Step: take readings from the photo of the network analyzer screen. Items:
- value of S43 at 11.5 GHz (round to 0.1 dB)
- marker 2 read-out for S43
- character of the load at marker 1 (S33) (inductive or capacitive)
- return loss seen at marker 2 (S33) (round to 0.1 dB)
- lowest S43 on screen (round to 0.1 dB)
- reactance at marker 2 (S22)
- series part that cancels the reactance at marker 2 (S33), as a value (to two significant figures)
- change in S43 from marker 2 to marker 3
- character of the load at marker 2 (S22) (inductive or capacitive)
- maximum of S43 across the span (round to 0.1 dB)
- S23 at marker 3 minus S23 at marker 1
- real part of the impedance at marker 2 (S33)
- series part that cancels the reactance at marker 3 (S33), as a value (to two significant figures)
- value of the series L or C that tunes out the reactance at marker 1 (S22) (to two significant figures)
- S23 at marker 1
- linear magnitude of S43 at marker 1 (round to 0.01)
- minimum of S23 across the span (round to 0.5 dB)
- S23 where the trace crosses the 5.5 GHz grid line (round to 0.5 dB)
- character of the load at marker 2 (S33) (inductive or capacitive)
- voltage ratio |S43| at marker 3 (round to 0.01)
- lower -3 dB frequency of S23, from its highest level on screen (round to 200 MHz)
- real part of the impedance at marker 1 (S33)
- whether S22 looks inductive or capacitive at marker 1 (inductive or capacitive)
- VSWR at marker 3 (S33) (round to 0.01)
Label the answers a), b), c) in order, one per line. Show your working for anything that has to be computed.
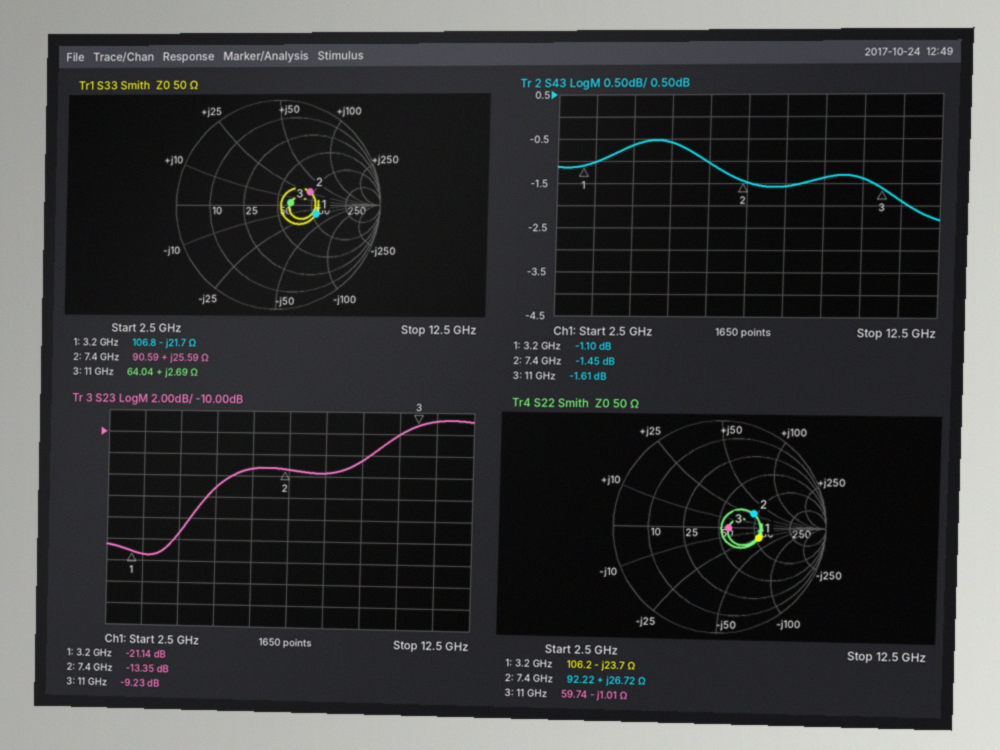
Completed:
a) -1.9 dB
b) -1.45 dB
c) capacitive
d) 9.5 dB
e) -2.3 dB
f) +26.72 Ω
g) C = 1/(2π × 7.4 GHz × 25.59 Ω) ≈ 840 fF
h) -1.61 − (-1.45) = -0.16 dB
i) inductive
j) -0.5 dB
k) -9.23 − (-21.14) = 11.91 dB
l) 90.59 Ω
m) C = 1/(2π × 11 GHz × 2.69 Ω) ≈ 5.4 pF
n) L = 23.7 Ω/(2π × 3.2 GHz) ≈ 1.2 nH
o) -21.14 dB
p) 10^(-1.1/20) ≈ 0.88
q) -21.5 dB
r) -15.0 dB
s) inductive
t) 10^(-1.61/20) ≈ 0.83
u) 9.8 GHz
v) 106.8 Ω
w) capacitive
x) 1.29
